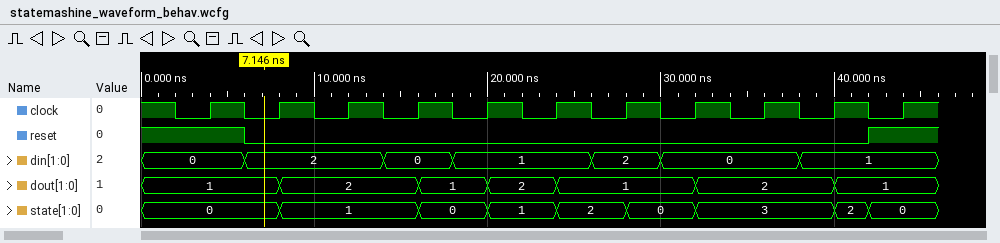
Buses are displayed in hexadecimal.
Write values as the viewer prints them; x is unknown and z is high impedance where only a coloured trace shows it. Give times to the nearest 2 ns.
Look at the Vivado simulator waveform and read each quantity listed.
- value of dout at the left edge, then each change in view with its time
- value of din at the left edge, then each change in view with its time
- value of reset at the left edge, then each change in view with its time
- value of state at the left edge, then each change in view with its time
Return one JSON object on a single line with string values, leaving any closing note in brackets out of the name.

{"value of dout at the left edge, then each change in view with its time": "1, 2 at 8 ns, 1 at 16 ns, 2 at 20 ns, 1 at 24 ns, 2 at 32 ns, 1 at 40 ns", "value of din at the left edge, then each change in view with its time": "0, 2 at 6 ns, 0 at 14 ns, 1 at 18 ns, 2 at 26 ns, 0 at 30 ns, 1 at 38 ns", "value of reset at the left edge, then each change in view with its time": "1, 0 at 6 ns, 1 at 42 ns", "value of state at the left edge, then each change in view with its time": "0, 1 at 8 ns, 0 at 16 ns, 1 at 20 ns, 2 at 24 ns, 0 at 28 ns, 3 at 32 ns, 2 at 40 ns, 0 at 42 ns"}
